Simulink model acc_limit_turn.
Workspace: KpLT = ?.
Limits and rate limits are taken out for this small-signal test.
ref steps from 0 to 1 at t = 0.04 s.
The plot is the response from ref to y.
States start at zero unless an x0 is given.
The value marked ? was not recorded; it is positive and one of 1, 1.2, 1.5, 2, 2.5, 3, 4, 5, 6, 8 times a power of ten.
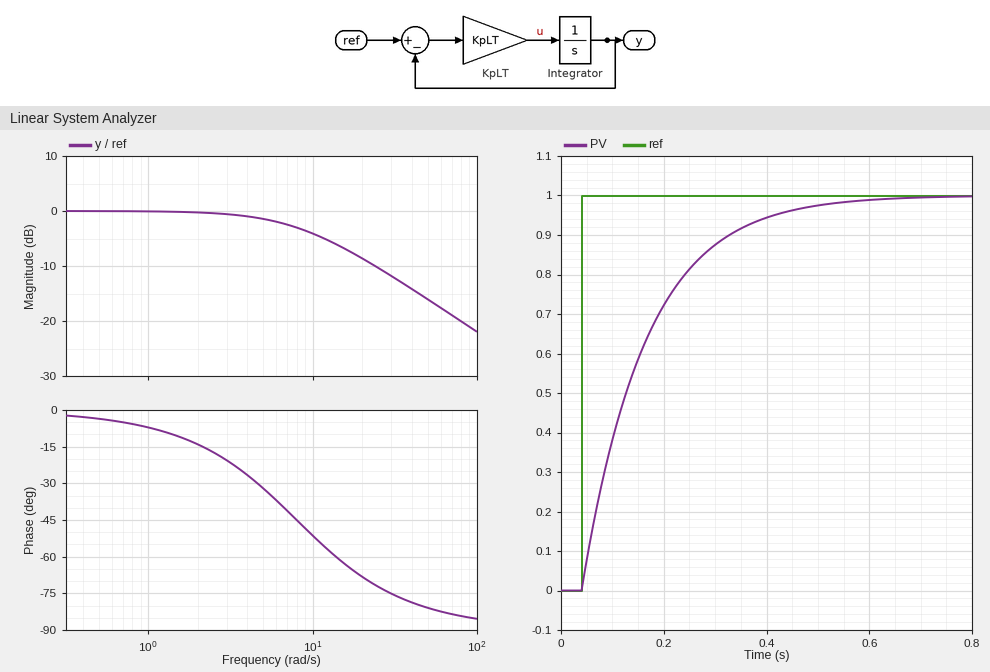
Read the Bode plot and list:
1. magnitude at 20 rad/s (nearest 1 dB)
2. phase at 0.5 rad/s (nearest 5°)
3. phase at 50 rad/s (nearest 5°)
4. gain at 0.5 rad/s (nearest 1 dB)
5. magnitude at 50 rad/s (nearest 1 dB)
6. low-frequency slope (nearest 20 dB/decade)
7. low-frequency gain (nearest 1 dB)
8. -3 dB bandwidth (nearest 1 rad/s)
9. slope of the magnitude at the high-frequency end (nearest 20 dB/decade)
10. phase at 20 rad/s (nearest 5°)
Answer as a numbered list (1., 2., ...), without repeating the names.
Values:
1. -9 dB
2. -5°
3. -80°
4. 0 dB
5. -16 dB
6. 0 dB/decade
7. 0 dB
8. 8 rad/s
9. -20 dB/decade
10. -70°
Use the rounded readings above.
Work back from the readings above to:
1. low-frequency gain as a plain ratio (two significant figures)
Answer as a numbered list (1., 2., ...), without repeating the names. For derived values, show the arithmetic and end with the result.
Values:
1. 10^(0 / 20) = 1.0
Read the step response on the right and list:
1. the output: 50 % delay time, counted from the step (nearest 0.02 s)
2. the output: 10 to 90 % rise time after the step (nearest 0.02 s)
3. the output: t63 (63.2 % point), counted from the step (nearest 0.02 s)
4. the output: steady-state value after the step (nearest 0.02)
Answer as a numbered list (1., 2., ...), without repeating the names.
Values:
1. 0.08 s
2. 0.28 s
3. 0.12 s
4. 1.00
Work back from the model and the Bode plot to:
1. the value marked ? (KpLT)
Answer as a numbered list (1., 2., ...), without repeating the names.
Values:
1. 8
